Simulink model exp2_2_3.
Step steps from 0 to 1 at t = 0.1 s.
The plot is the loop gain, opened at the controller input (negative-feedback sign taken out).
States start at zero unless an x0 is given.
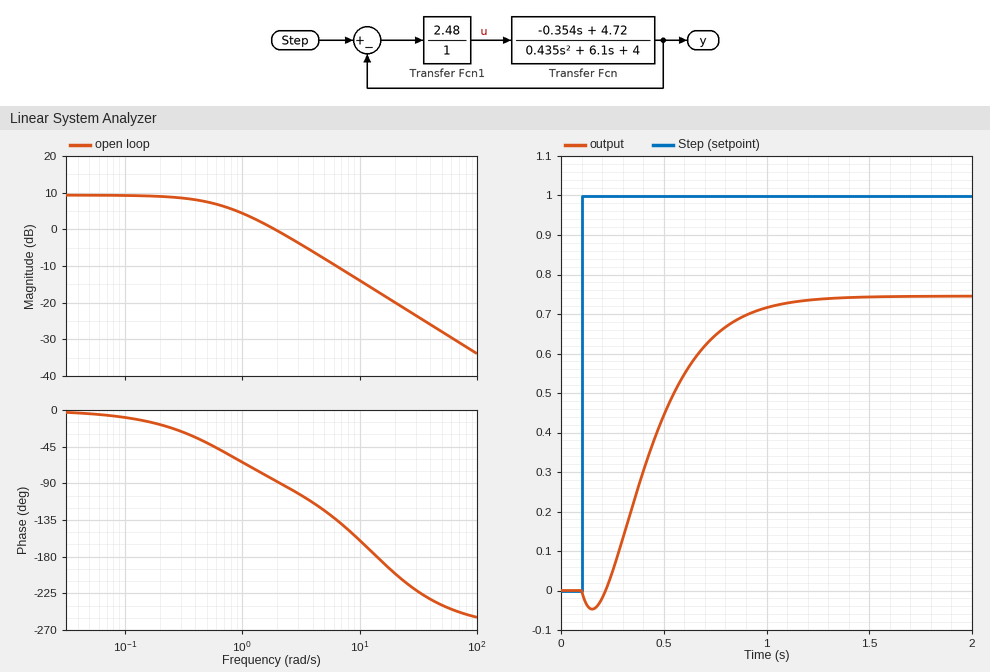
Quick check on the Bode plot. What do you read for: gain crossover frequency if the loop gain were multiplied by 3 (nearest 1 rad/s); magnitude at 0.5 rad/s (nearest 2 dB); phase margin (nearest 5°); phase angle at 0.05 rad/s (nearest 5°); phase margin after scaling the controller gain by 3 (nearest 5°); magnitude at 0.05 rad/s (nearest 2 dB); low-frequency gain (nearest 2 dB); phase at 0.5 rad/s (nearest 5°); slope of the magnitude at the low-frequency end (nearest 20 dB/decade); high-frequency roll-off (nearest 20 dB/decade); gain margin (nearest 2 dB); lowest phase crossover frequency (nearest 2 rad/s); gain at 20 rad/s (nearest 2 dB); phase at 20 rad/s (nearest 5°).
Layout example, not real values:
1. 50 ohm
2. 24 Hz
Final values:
1. 6 rad/s
2. 8 dB
3. 95°
4. -5°
5. 50°
6. 10 dB
7. 10 dB
8. -40°
9. 0 dB/decade
10. -20 dB/decade
11. 16 dB
12. 14 rad/s
13. -20 dB
14. -200°
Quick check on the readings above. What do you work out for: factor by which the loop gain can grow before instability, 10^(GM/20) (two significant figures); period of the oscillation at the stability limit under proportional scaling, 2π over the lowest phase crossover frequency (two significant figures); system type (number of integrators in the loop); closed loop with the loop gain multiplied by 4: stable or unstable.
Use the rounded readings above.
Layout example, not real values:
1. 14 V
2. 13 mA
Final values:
1. 6.3
2. 0.45 s
3. 0
4. stable
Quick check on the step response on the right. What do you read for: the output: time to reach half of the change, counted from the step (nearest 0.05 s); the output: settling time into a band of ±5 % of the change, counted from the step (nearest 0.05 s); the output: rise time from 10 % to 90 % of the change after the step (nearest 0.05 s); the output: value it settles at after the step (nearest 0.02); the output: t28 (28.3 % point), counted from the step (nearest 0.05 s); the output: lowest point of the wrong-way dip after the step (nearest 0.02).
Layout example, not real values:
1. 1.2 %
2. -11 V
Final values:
1. 0.35 s
2. 0.85 s
3. 0.55 s
4. 0.74
5. 0.25 s
6. -0.04
